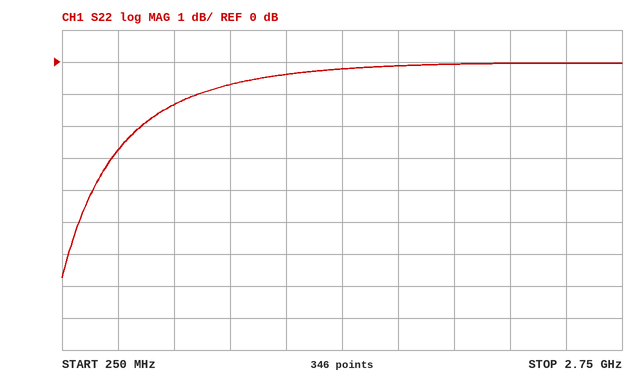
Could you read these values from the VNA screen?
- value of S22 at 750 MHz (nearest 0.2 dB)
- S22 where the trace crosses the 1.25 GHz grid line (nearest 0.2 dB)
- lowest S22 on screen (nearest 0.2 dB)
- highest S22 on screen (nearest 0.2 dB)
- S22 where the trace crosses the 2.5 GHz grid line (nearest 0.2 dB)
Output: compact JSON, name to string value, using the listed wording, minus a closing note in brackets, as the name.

{"value of S22 at 750 MHz": "-1.4 dB", "S22 where the trace crosses the 1.25 GHz grid line": "-0.4 dB", "lowest S22 on screen": "-6.8 dB", "highest S22 on screen": "0.0 dB", "S22 where the trace crosses the 2.5 GHz grid line": "0.0 dB"}
